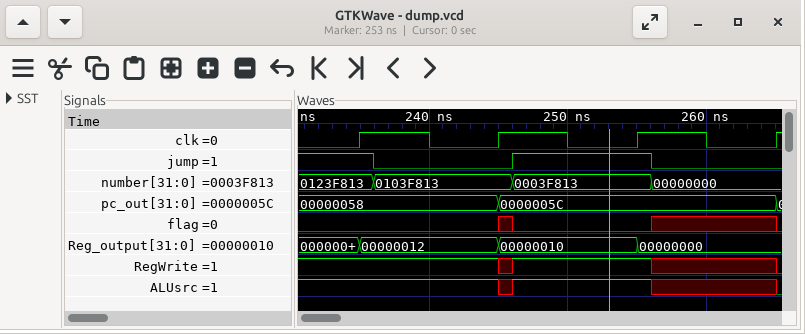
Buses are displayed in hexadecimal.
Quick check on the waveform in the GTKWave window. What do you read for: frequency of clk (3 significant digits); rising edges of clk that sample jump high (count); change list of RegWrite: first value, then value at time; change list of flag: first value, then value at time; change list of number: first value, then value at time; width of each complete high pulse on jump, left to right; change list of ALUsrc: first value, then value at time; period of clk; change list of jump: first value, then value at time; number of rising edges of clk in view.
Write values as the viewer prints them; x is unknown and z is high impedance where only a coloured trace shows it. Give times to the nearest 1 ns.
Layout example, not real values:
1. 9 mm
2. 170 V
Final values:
1. 100 MHz
2. 2
3. 1, x at 245 ns, 1 at 246 ns, x at 256 ns, 0 at 265 ns
4. 0, x at 245 ns, 0 at 246 ns, x at 256 ns, 0 at 265 ns
5. 0123F813, 0103F813 at 236 ns, 0003F813 at 246 ns, 00000000 at 256 ns
6. 10 ns
7. 1, x at 245 ns, 1 at 246 ns, x at 256 ns, 0 at 265 ns
8. 10 ns
9. 1, 0 at 236 ns, 1 at 246 ns, 0 at 256 ns
10. 4
